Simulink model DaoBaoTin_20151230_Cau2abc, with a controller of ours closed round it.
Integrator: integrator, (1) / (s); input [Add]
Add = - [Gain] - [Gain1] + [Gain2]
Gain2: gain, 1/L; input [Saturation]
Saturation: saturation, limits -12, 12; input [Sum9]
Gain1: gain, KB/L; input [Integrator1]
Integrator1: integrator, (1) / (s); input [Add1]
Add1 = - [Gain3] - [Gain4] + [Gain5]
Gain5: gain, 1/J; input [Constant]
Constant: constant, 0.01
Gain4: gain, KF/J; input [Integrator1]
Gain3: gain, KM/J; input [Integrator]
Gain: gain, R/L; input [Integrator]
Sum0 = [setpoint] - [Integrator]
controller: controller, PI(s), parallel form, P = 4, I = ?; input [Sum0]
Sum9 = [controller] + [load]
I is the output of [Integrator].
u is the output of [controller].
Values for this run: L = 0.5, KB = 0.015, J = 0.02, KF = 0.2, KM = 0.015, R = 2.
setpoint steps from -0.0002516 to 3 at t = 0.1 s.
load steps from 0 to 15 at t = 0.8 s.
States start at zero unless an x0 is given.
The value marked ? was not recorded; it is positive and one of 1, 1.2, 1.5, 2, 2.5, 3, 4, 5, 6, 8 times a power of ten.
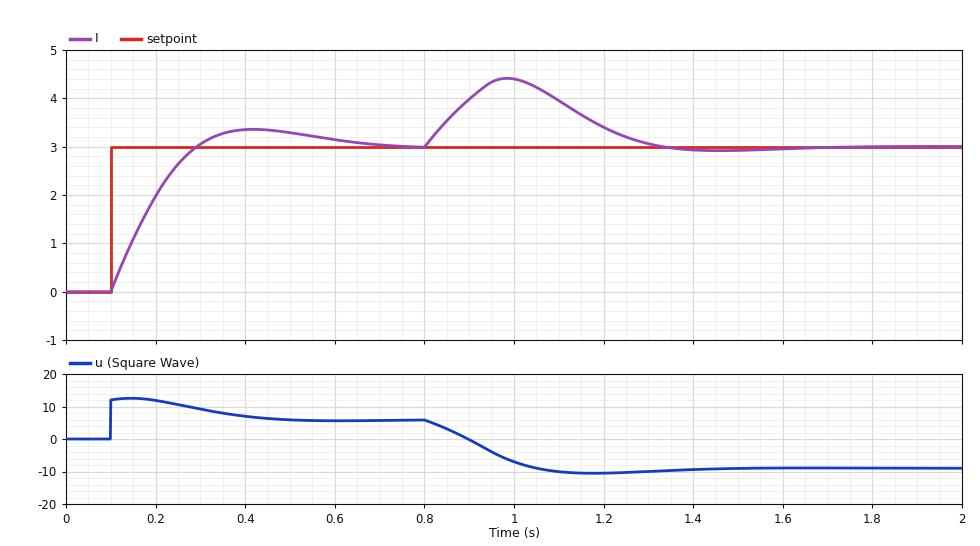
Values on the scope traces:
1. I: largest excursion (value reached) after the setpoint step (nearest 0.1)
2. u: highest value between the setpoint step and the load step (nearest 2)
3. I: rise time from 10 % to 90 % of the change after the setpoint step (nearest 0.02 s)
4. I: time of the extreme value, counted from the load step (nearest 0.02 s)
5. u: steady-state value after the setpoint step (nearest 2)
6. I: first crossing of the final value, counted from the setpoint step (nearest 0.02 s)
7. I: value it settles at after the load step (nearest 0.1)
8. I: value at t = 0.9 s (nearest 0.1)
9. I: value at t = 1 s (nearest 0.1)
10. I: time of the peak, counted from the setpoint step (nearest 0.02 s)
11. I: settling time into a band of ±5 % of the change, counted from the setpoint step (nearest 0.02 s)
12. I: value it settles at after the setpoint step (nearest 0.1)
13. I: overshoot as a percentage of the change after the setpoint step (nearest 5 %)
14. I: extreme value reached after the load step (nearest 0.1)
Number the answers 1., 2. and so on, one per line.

1. 3.4
2. 12
3. 0.14 s
4. 0.18 s
5. 6
6. 0.20 s
7. 3.0
8. 4.0
9. 4.4
10. 0.32 s
11. 0.50 s
12. 3.0
13. 10 %
14. 4.4
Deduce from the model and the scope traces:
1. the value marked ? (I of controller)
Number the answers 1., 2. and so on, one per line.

1. 40
